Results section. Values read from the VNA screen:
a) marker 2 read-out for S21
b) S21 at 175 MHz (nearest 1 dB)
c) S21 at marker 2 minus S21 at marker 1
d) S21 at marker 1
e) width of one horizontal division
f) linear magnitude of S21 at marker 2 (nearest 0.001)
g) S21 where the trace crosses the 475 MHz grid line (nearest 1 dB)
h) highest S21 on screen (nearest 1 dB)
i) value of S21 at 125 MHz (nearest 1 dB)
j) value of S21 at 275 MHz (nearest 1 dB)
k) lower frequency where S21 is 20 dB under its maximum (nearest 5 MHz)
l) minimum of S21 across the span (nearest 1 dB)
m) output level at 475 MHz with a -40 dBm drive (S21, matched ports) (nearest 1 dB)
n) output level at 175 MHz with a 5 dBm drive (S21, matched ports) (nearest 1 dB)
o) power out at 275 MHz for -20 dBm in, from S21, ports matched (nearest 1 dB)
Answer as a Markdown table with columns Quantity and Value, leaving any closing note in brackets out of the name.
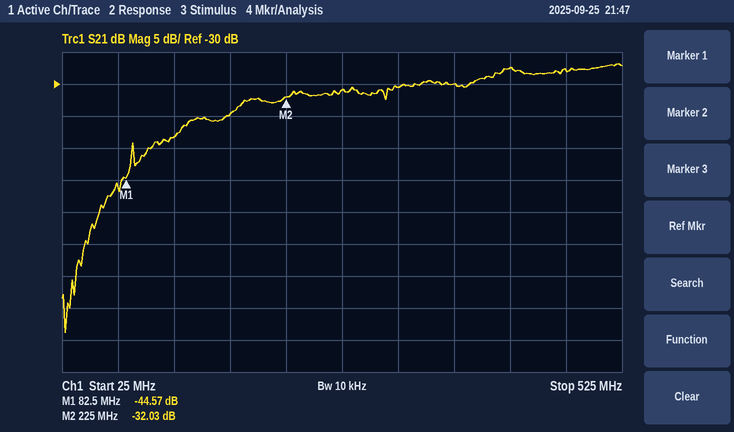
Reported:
| Quantity | Value |
|---|---|
| marker 2 read-out for S21 | -32.03 dB |
| S21 at 175 MHz | -35 dB |
| S21 at marker 2 minus S21 at marker 1 | 12.54 dB |
| S21 at marker 1 | -44.57 dB |
| width of one horizontal division | 50 MHz |
| linear magnitude of S21 at marker 2 | 0.025 |
| S21 where the trace crosses the 475 MHz grid line | -28 dB |
| highest S21 on screen | -27 dB |
| value of S21 at 125 MHz | -38 dB |
| value of S21 at 275 MHz | -31 dB |
| lower frequency where S21 is 20 dB under its maximum | 70 MHz |
| minimum of S21 across the span | -69 dB |
| output level at 475 MHz with a -40 dBm drive (S21, matched ports) | -68 dBm |
| output level at 175 MHz with a 5 dBm drive (S21, matched ports) | -30 dBm |
| power out at 275 MHz for -20 dBm in, from S21, ports matched | -51 dBm |
